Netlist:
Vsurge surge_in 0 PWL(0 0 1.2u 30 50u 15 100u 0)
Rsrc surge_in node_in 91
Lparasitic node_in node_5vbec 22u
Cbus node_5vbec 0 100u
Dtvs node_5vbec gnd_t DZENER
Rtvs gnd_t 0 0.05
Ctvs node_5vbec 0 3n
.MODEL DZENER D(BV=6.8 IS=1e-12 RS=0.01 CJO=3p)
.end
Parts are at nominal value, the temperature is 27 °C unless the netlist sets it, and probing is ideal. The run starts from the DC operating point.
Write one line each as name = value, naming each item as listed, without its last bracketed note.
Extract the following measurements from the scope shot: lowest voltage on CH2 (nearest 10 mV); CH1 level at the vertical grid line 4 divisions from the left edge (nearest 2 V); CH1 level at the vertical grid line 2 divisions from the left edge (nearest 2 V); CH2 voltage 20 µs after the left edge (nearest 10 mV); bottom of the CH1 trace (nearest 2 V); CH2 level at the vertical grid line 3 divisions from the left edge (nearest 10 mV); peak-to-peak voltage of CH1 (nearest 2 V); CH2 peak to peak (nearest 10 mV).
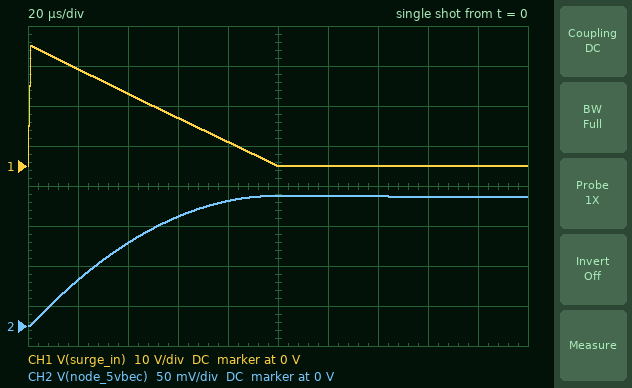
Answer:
lowest voltage on CH2 = 0 V
CH1 level at the vertical grid line 4 divisions from the left edge = 6 V
CH1 level at the vertical grid line 2 divisions from the left edge = 18 V
CH2 voltage 20 µs after the left edge = 60 mV
bottom of the CH1 trace = 0 V
CH2 level at the vertical grid line 3 divisions from the left edge = 140 mV
peak-to-peak voltage of CH1 = 30 V
CH2 peak to peak = 160 mV
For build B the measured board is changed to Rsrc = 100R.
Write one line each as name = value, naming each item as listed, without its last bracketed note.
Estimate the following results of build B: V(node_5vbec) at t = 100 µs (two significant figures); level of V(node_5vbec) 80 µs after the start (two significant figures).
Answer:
V(node_5vbec) at t = 100 µs = 150 mV
level of V(node_5vbec) 80 µs after the start = 140 mV
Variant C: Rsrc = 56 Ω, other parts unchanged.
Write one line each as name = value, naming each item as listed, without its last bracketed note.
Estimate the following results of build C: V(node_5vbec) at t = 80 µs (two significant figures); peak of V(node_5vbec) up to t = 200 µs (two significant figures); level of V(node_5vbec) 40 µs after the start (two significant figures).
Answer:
V(node_5vbec) at t = 80 µs = 250 mV
peak of V(node_5vbec) up to t = 200 µs = 260 mV
level of V(node_5vbec) 40 µs after the start = 170 mV
